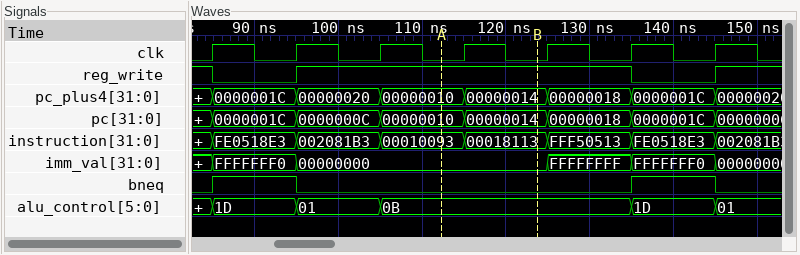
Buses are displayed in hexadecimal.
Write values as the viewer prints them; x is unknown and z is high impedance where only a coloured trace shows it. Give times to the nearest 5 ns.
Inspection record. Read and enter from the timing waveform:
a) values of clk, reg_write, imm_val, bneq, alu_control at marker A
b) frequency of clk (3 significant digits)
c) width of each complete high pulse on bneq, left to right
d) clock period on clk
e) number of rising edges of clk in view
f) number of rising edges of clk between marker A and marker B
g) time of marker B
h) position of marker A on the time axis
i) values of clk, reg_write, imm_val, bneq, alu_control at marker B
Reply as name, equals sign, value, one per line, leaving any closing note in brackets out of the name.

values of clk, reg_write, imm_val, bneq, alu_control at marker A = clk=0, reg_write=1, imm_val=00000000, bneq=0, alu_control=0B
frequency of clk = 100 MHz
width of each complete high pulse on bneq, left to right = 10 ns, 10 ns
clock period on clk = 10 ns
number of rising edges of clk in view = 7
number of rising edges of clk between marker A and marker B = 1
time of marker B = 125 ns
position of marker A on the time axis = 110 ns
values of clk, reg_write, imm_val, bneq, alu_control at marker B = clk=0, reg_write=1, imm_val=00000000, bneq=0, alu_control=0B
